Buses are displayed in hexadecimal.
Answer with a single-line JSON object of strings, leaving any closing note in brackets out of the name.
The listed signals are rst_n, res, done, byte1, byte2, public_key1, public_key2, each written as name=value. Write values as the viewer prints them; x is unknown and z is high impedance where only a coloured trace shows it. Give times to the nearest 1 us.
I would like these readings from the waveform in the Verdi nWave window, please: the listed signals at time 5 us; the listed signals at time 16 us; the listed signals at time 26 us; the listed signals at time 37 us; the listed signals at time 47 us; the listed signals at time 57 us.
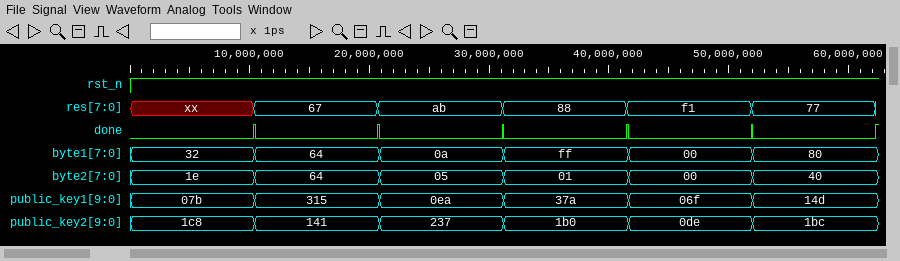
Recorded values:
{"the listed signals at time 5 us": "rst_n=1, res=xx, done=0, byte1=32, byte2=1e, public_key1=07b, public_key2=1c8", "the listed signals at time 16 us": "rst_n=1, res=67, done=0, byte1=64, byte2=64, public_key1=315, public_key2=141", "the listed signals at time 26 us": "rst_n=1, res=ab, done=0, byte1=0a, byte2=05, public_key1=0ea, public_key2=237", "the listed signals at time 37 us": "rst_n=1, res=88, done=0, byte1=ff, byte2=01, public_key1=37a, public_key2=1b0", "the listed signals at time 47 us": "rst_n=1, res=f1, done=0, byte1=00, byte2=00, public_key1=06f, public_key2=0de", "the listed signals at time 57 us": "rst_n=1, res=77, done=0, byte1=80, byte2=40, public_key1=14d, public_key2=1bc"}
